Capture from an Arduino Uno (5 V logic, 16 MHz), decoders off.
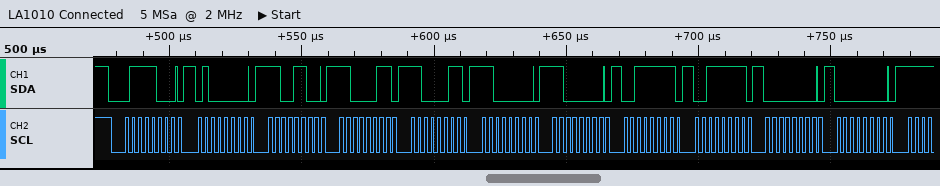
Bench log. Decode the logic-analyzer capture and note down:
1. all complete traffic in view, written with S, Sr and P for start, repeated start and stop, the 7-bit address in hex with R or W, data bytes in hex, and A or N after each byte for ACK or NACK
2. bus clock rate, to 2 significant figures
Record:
S 3CW A 40 A CC A C3 A C3 A C0 A C0 A 3F A 3F A 00 A 00 A
400 kHz
